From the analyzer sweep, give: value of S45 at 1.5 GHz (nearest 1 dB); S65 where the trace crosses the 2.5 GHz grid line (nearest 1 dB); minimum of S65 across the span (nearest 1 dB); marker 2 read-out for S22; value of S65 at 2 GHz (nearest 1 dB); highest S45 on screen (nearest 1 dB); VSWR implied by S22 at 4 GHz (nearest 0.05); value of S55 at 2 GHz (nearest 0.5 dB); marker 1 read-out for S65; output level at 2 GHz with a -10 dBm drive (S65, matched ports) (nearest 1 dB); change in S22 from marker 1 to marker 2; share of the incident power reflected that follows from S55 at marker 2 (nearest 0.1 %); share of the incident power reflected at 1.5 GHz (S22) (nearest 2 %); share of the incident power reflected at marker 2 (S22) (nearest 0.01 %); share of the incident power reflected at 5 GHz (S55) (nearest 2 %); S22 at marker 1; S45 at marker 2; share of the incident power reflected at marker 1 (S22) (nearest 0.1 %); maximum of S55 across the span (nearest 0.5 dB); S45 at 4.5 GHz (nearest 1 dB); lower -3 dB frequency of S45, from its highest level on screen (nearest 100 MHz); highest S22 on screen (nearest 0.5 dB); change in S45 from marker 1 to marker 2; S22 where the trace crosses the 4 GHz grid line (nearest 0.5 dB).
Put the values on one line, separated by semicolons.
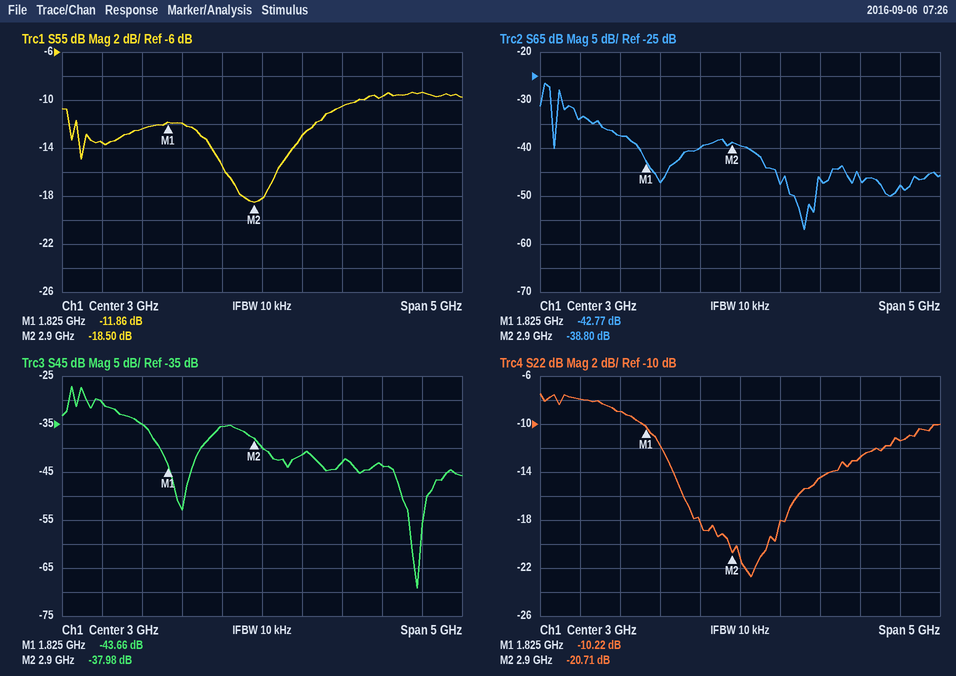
-35 dB; -40 dB; -57 dB; -20.71 dB; -47 dB; -27 dB; 1.45; -12.0 dB; -42.77 dB; -57 dBm; -10.49 dB; 1.4 %; 12 %; 0.85 %; 12 %; -10.22 dB; -37.98 dB; 9.5 %; -9.5 dB; -44 dB; 600 MHz; -7.5 dB; 5.68 dB; -14.5 dB
